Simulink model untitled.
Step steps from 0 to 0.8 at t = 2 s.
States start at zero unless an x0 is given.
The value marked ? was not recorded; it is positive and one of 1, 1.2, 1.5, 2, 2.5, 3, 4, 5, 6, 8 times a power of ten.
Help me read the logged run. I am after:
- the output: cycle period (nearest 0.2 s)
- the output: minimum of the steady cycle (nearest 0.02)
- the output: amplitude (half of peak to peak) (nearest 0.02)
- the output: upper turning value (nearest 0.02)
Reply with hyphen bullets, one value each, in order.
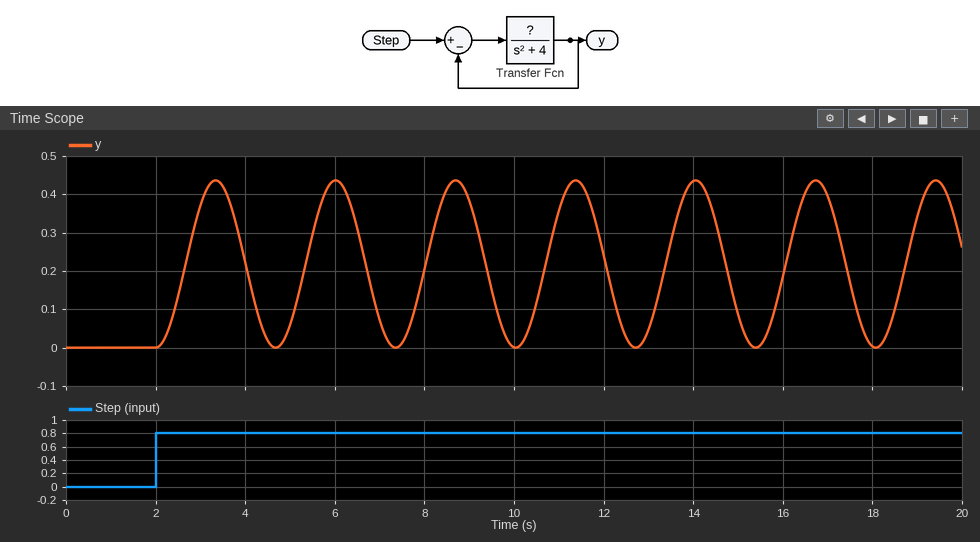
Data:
- 2.6 s
- 0.00
- 0.22
- 0.44
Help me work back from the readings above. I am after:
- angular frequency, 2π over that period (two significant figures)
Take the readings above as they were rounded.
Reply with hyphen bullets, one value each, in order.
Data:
- 2.4 rad/s
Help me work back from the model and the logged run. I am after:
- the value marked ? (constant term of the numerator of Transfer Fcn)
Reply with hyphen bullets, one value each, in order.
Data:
- 1.5
